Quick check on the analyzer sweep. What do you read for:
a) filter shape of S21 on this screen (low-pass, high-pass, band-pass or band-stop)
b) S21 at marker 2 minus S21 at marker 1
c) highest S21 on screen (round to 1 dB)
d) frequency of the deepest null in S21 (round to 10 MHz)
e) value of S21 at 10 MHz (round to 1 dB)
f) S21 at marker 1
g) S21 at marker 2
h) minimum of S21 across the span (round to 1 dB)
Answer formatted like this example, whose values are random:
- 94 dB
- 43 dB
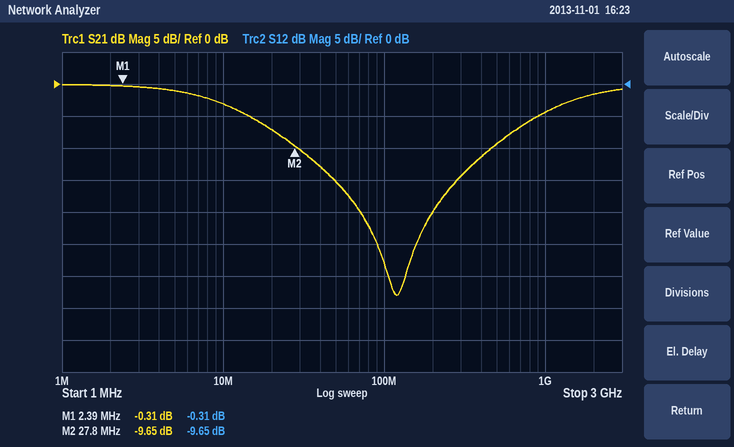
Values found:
- band-stop
- -9.34 dB
- 0 dB
- 120 MHz
- -3 dB
- -0.31 dB
- -9.65 dB
- -33 dB
